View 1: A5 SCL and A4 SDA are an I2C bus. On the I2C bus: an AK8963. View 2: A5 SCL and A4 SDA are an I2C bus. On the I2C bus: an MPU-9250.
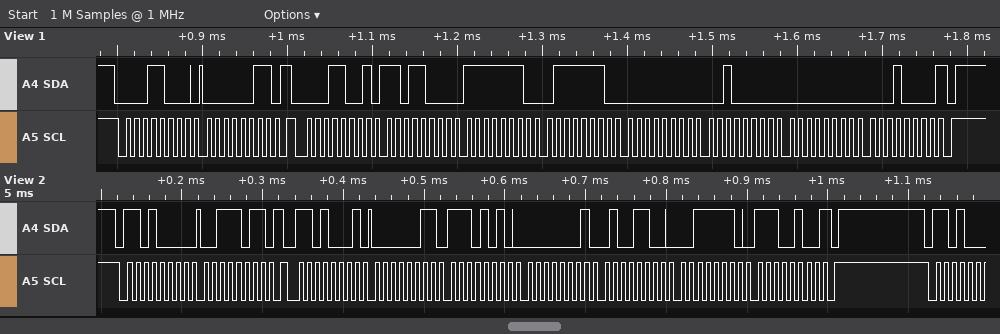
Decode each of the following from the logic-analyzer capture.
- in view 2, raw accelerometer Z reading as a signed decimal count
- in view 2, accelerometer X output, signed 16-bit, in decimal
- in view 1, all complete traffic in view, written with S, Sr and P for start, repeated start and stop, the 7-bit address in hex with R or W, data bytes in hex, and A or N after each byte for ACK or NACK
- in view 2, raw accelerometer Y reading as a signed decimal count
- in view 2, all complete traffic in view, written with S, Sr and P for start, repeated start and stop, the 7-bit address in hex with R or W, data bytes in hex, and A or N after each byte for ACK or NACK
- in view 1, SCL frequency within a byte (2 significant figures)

16100
1002
S 0CW A 03 A Sr 0CR A D8 A FE A 7E A 00 A 20 A 00 A 10 N P
332
S 68W A 3B A Sr 68R A 03 A EA A 01 A 4C A 3E A E4 N P
100 kHz
